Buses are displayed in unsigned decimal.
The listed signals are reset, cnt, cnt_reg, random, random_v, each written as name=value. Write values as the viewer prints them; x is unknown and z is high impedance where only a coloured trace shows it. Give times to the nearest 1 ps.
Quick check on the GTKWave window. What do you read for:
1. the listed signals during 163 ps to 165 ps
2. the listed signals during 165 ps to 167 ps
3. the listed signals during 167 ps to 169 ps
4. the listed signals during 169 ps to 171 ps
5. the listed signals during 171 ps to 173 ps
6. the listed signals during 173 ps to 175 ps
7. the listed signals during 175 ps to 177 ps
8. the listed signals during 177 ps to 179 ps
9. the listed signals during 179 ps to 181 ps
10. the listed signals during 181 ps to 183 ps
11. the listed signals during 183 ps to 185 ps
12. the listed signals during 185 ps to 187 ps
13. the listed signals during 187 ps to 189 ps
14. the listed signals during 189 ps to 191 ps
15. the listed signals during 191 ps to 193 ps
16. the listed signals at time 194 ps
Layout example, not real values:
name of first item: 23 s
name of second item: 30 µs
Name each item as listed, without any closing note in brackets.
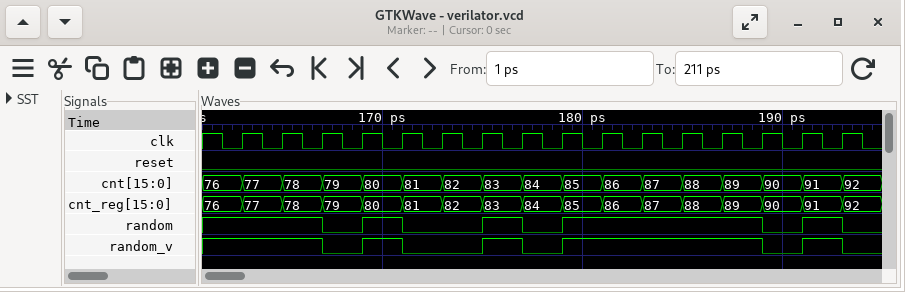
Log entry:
the listed signals during 163 ps to 165 ps: reset=0, cnt=77, cnt_reg=77, random=1, random_v=1
the listed signals during 165 ps to 167 ps: reset=0, cnt=78, cnt_reg=78, random=1, random_v=1
the listed signals during 167 ps to 169 ps: reset=0, cnt=79, cnt_reg=79, random=0, random_v=0
the listed signals during 169 ps to 171 ps: reset=0, cnt=80, cnt_reg=80, random=1, random_v=1
the listed signals during 171 ps to 173 ps: reset=0, cnt=81, cnt_reg=81, random=0, random_v=0
the listed signals during 173 ps to 175 ps: reset=0, cnt=82, cnt_reg=82, random=0, random_v=0
the listed signals during 175 ps to 177 ps: reset=0, cnt=83, cnt_reg=83, random=1, random_v=1
the listed signals during 177 ps to 179 ps: reset=0, cnt=84, cnt_reg=84, random=0, random_v=0
the listed signals during 179 ps to 181 ps: reset=0, cnt=85, cnt_reg=85, random=1, random_v=1
the listed signals during 181 ps to 183 ps: reset=0, cnt=86, cnt_reg=86, random=1, random_v=1
the listed signals during 183 ps to 185 ps: reset=0, cnt=87, cnt_reg=87, random=1, random_v=1
the listed signals during 185 ps to 187 ps: reset=0, cnt=88, cnt_reg=88, random=1, random_v=1
the listed signals during 187 ps to 189 ps: reset=0, cnt=89, cnt_reg=89, random=1, random_v=1
the listed signals during 189 ps to 191 ps: reset=0, cnt=90, cnt_reg=90, random=0, random_v=0
the listed signals during 191 ps to 193 ps: reset=0, cnt=91, cnt_reg=91, random=1, random_v=1
the listed signals at time 194 ps: reset=0, cnt=92, cnt_reg=92, random=0, random_v=0
